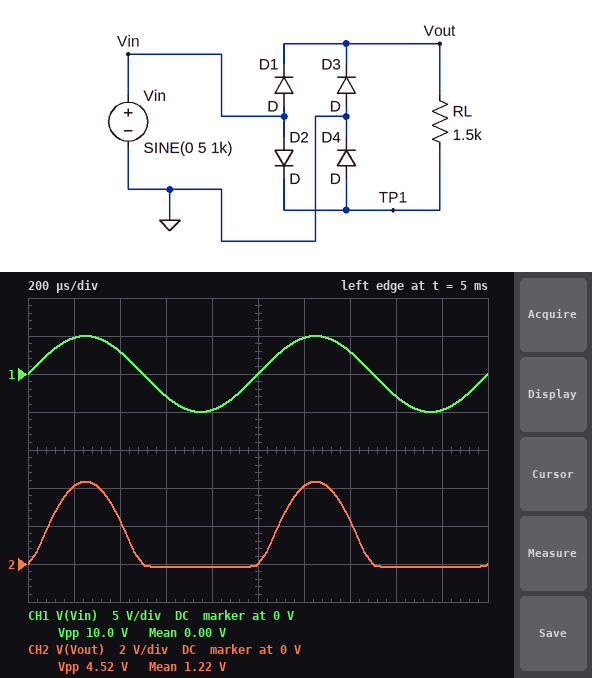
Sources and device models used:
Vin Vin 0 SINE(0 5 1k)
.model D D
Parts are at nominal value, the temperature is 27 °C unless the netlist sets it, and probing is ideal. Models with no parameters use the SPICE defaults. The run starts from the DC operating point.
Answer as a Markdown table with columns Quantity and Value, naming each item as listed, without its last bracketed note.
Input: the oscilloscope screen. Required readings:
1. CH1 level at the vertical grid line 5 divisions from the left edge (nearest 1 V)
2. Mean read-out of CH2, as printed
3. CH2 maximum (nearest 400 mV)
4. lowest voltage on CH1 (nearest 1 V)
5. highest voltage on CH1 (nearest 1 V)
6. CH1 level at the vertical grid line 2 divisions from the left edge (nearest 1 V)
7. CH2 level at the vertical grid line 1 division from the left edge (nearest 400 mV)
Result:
| Quantity | Value |
|---|---|
| CH1 level at the vertical grid line 5 divisions from the left edge | 0 V |
| Mean read-out of CH2, as printed | 1.22 V |
| CH2 maximum | 4.4 V |
| lowest voltage on CH1 | -5 V |
| highest voltage on CH1 | 5 V |
| CH1 level at the vertical grid line 2 divisions from the left edge | 3 V |
| CH2 level at the vertical grid line 1 division from the left edge | 4.0 V |
